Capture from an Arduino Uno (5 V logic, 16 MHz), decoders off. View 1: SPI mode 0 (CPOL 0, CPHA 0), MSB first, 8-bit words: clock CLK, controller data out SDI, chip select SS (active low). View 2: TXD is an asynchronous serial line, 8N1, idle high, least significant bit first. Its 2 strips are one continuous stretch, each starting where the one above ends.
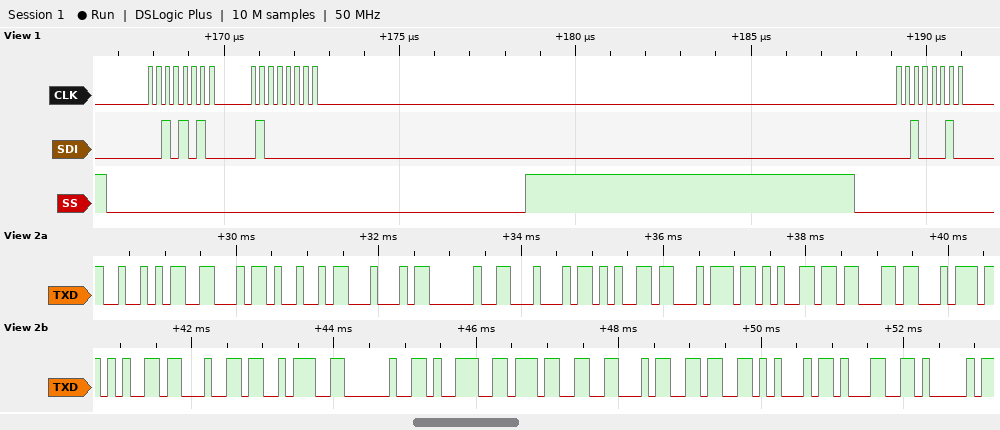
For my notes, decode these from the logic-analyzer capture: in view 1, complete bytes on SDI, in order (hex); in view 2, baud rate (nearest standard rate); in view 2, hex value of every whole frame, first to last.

2A 40 22
9600 baud
0x52 0x46 0x49 0x44 0x20 0x44 0x65 0x74 0x65 0x63 0x74 0x65 0x64 0x3A 0x20 0x39 0x37 0x46 0x36 0x45 0x31 0x41
